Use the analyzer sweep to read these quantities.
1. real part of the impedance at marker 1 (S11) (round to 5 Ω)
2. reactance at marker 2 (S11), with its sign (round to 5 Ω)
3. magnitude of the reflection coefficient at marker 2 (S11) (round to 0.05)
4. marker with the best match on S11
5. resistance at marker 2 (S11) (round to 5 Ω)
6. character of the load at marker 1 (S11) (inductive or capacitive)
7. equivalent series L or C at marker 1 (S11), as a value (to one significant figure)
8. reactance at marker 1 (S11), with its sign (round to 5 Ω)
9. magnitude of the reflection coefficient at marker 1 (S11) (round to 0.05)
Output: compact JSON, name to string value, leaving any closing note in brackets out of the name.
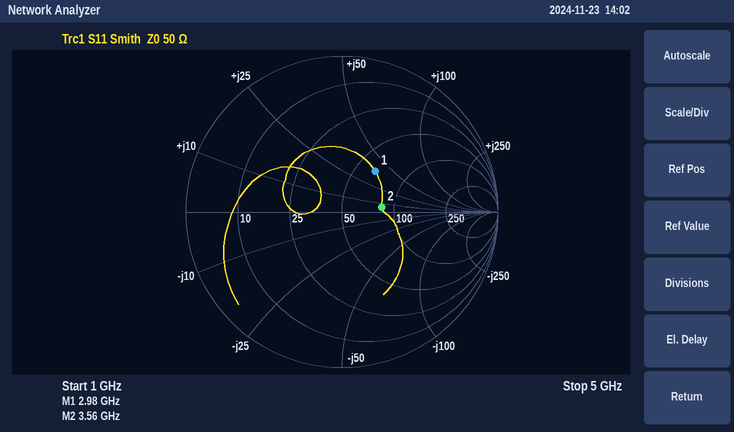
{"real part of the impedance at marker 1 (S11)": "65 Ω", "reactance at marker 2 (S11), with its sign": "+5 Ω", "magnitude of the reflection coefficient at marker 2 (S11)": "0.25", "marker with the best match on S11": "marker 2", "resistance at marker 2 (S11)": "85 Ω", "character of the load at marker 1 (S11)": "inductive", "equivalent series L or C at marker 1 (S11), as a value": "2 nH", "reactance at marker 1 (S11), with its sign": "+40 Ω", "magnitude of the reflection coefficient at marker 1 (S11)": "0.35"}
